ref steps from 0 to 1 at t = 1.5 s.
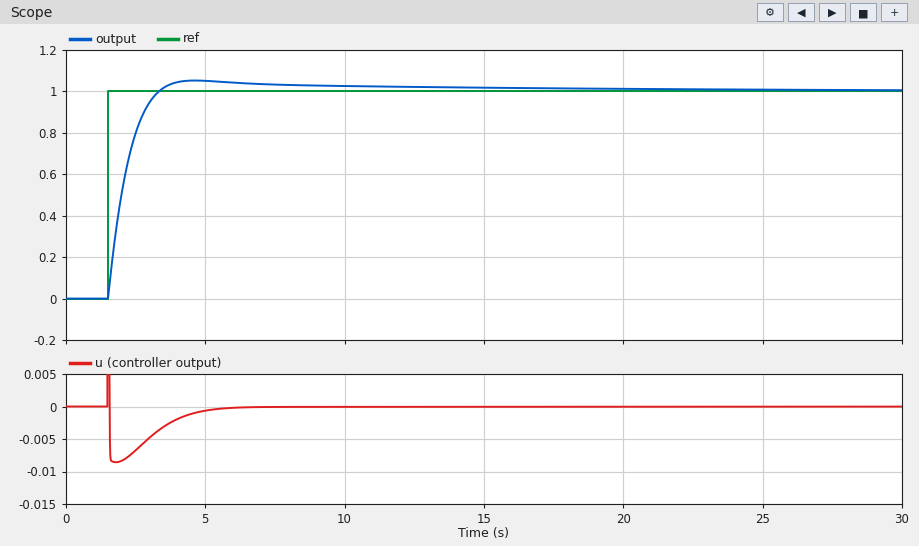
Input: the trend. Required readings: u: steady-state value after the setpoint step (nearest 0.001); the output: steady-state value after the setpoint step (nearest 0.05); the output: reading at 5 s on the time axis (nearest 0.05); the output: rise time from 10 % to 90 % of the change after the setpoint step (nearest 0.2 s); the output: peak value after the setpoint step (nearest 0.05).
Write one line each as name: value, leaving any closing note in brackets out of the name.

u: steady-state value after the setpoint step: 0.000
the output: steady-state value after the setpoint step: 1.00
the output: reading at 5 s on the time axis: 1.05
the output: rise time from 10 % to 90 % of the change after the setpoint step: 1.2 s
the output: peak value after the setpoint step: 1.05
